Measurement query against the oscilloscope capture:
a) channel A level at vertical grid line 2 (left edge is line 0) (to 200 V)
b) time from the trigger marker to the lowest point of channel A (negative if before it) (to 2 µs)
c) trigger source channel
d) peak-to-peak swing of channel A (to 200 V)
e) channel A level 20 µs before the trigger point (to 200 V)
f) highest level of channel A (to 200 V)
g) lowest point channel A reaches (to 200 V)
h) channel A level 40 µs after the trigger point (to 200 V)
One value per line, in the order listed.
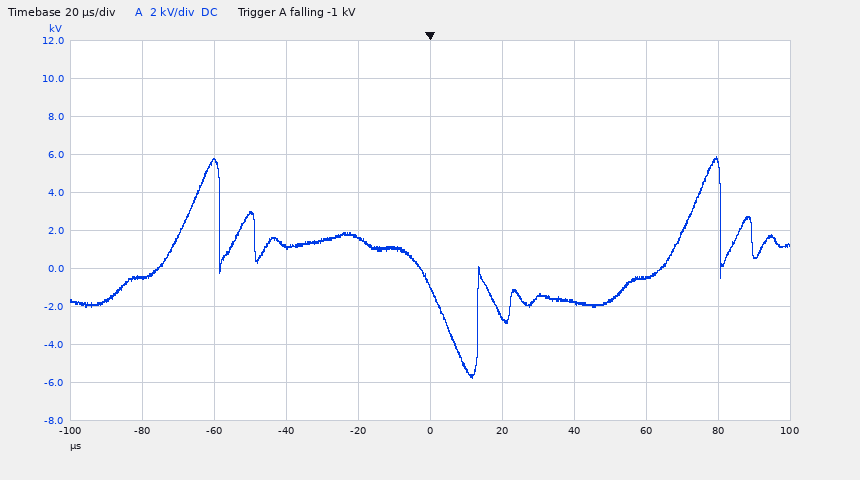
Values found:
5.6 kV
+12 µs
channel A
11.6 kV
1.6 kV
5.8 kV
-5.8 kV
-1.8 kV
